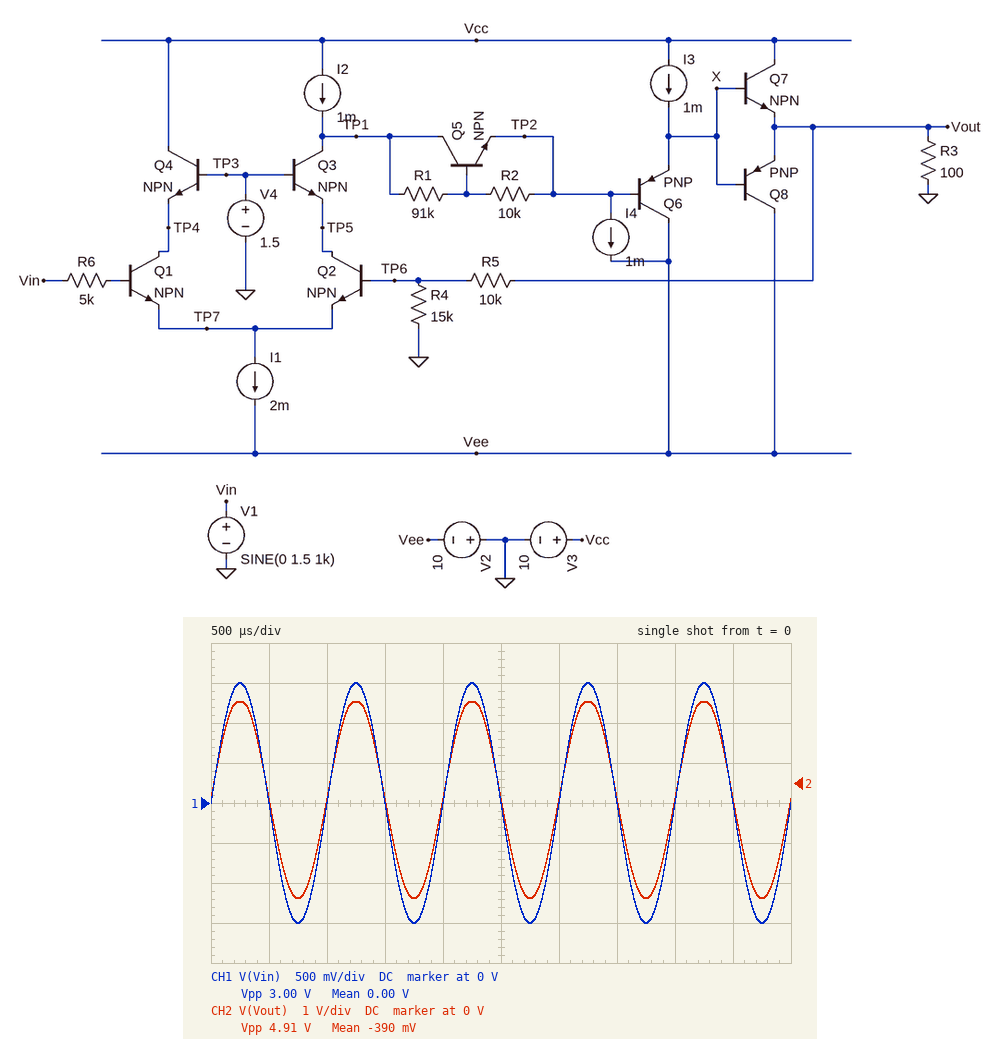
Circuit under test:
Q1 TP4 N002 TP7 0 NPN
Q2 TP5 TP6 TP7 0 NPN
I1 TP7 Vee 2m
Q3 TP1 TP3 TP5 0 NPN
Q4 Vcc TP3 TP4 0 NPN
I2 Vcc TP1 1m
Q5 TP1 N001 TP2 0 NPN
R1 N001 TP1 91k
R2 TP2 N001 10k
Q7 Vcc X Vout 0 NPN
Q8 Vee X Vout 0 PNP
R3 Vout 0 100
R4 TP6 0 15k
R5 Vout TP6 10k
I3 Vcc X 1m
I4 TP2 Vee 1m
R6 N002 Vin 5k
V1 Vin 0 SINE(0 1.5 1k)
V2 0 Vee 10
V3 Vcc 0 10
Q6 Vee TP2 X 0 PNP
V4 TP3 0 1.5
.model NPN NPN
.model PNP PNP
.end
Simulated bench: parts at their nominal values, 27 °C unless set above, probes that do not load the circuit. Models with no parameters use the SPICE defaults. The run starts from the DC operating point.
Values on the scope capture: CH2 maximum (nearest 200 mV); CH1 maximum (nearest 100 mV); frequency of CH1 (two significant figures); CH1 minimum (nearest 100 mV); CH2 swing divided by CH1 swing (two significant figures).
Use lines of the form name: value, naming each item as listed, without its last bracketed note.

CH2 maximum: 2.0 V
CH1 maximum: 1.5 V
frequency of CH1: 1.0 kHz
CH1 minimum: -1.5 V
CH2 swing divided by CH1 swing: 1.6
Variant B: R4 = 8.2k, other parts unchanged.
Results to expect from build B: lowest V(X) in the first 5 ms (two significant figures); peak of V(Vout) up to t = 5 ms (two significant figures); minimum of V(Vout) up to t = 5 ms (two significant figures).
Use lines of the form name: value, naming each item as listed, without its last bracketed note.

lowest V(X) in the first 5 ms: -4.7 V
peak of V(Vout) up to t = 5 ms: 2.7 V
minimum of V(Vout) up to t = 5 ms: -3.8 V
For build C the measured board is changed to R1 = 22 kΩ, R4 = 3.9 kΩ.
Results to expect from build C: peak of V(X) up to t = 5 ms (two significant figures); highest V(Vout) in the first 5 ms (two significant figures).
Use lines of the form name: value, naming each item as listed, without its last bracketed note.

peak of V(X) up to t = 5 ms: 5.2 V
highest V(Vout) in the first 5 ms: 4.3 V
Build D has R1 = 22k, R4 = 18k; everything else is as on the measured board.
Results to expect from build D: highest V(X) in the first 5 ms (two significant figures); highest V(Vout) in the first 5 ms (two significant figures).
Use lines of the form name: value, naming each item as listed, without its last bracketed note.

highest V(X) in the first 5 ms: 2.7 V
highest V(Vout) in the first 5 ms: 1.9 V
